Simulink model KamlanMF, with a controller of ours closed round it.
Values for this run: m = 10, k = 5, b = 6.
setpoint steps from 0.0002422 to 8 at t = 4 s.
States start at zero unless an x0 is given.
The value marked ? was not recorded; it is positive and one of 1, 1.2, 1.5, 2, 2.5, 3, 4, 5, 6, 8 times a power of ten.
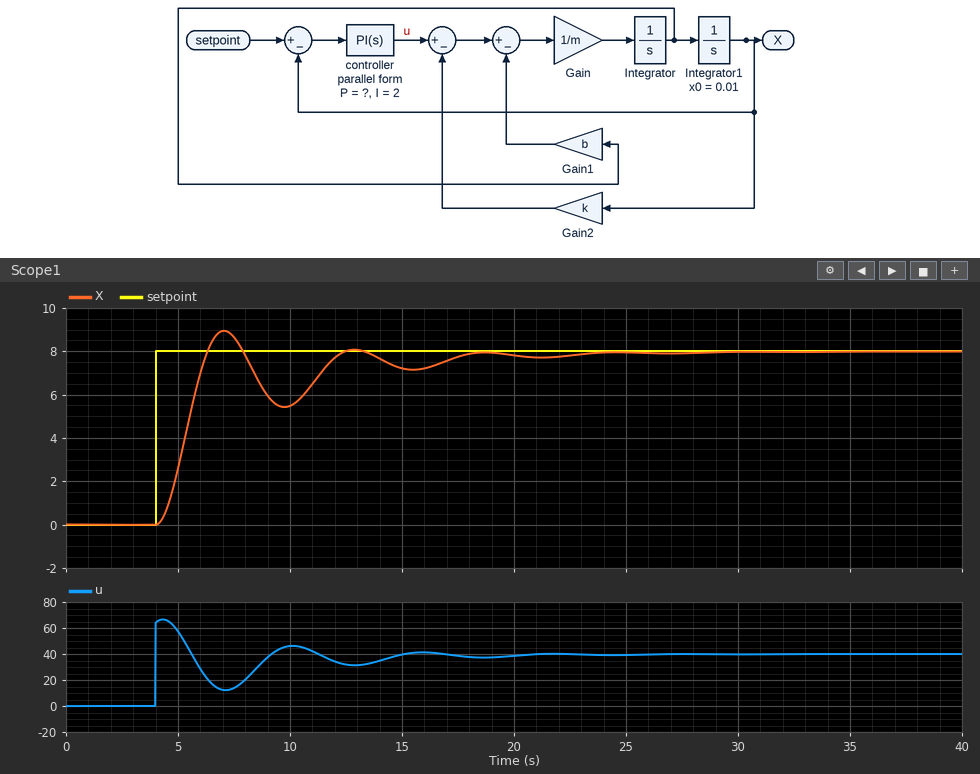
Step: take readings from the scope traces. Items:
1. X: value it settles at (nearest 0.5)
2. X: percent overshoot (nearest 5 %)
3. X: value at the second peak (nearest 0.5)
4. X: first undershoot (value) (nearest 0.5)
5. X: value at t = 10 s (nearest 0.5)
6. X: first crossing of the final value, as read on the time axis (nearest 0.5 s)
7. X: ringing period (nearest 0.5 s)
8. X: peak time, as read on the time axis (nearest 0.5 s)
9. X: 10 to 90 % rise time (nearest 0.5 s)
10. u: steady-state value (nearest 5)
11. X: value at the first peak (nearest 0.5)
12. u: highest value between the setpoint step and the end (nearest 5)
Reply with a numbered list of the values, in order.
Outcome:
1. 8.0
2. 10 %
3. 8.0
4. 5.5
5. 5.5
6. 6.5 s
7. 6.0 s
8. 7.0 s
9. 1.5 s
10. 40
11. 9.0
12. 65
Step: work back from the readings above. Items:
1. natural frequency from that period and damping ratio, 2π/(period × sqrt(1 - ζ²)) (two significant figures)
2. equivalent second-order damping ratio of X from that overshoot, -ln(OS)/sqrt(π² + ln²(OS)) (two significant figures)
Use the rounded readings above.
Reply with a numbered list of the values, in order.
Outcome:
1. 1.3 rad/s
2. 0.59
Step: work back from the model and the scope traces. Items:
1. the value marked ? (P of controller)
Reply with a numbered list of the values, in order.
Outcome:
1. 8
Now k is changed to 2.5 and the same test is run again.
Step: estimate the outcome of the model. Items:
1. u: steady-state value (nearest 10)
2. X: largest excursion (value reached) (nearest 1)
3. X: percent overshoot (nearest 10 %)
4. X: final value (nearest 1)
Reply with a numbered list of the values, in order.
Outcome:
1. 20
2. 11
3. 30 %
4. 8
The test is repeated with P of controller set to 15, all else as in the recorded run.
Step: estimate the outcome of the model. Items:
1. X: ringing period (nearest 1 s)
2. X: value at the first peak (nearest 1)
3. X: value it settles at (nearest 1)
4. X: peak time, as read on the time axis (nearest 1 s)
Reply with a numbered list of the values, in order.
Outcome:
1. 5 s
2. 10
3. 8
4. 6 s
